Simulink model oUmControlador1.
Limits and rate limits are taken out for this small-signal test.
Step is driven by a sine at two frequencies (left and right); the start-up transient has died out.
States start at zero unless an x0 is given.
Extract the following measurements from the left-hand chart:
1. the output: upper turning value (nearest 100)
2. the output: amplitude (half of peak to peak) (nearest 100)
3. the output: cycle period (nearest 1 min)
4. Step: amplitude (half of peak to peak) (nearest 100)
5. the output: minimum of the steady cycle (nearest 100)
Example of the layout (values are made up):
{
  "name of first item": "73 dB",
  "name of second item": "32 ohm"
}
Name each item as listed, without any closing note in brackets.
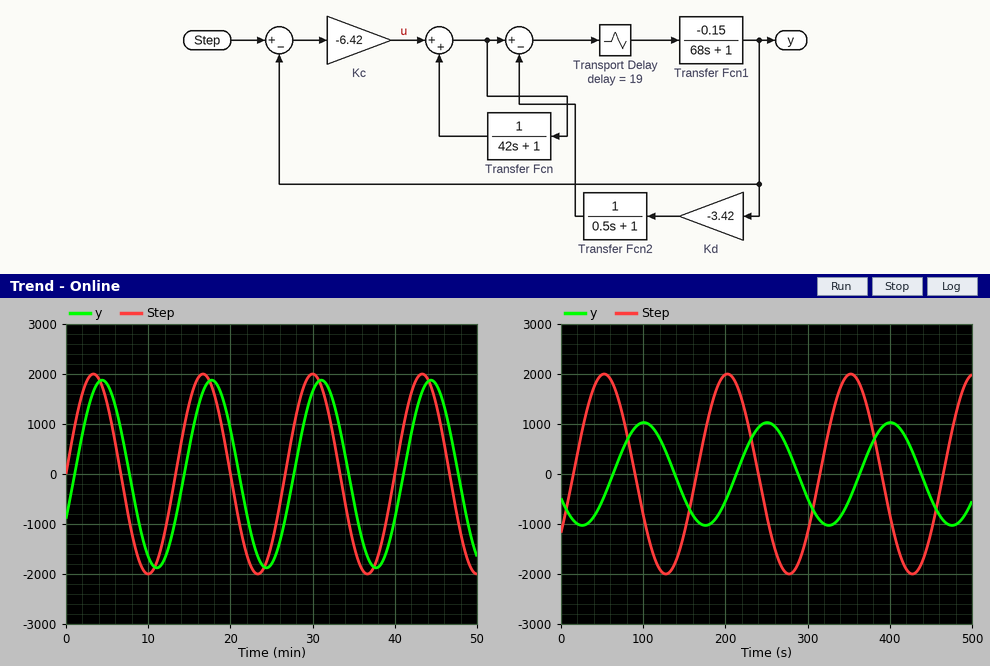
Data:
{
  "the output: upper turning value": "1900",
  "the output: amplitude (half of peak to peak)": "1900",
  "the output: cycle period": "13 min",
  "Step: amplitude (half of peak to peak)": "2000",
  "the output: minimum of the steady cycle": "-1900"
}
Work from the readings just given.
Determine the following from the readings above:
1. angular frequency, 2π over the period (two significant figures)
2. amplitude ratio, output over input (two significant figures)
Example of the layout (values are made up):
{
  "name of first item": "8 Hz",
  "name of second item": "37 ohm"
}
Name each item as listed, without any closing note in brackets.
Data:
{
  "angular frequency, 2π over the period": "0.48 rad/min",
  "amplitude ratio, output over input": "0.95"
}
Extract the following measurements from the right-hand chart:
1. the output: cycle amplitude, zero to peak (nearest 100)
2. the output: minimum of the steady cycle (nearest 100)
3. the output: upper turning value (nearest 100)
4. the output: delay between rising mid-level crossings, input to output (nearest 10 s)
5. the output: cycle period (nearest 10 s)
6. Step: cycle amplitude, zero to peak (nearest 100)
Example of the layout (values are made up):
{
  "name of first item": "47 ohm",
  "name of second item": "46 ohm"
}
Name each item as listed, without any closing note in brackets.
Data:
{
  "the output: cycle amplitude, zero to peak": "1000",
  "the output: minimum of the steady cycle": "-1000",
  "the output: upper turning value": "1000",
  "the output: delay between rising mid-level crossings, input to output": "50 s",
  "the output: cycle period": "150 s",
  "Step: cycle amplitude, zero to peak": "2000"
}
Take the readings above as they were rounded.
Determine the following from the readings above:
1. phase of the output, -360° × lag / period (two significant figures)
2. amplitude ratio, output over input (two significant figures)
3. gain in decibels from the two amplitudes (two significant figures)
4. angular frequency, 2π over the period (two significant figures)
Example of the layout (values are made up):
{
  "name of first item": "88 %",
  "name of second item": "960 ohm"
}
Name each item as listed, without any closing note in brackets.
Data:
{
  "phase of the output, -360° × lag / period": "-120°",
  "amplitude ratio, output over input": "0.50",
  "gain in decibels from the two amplitudes": "-6.0 dB",
  "angular frequency, 2π over the period": "0.042 rad/s"
}
